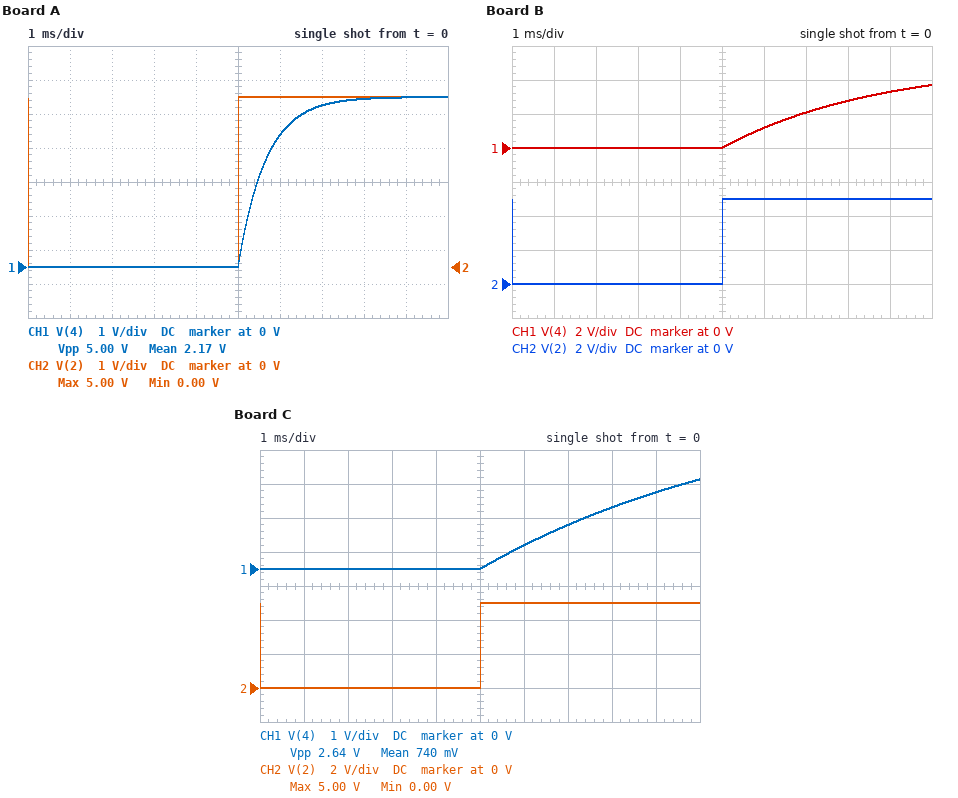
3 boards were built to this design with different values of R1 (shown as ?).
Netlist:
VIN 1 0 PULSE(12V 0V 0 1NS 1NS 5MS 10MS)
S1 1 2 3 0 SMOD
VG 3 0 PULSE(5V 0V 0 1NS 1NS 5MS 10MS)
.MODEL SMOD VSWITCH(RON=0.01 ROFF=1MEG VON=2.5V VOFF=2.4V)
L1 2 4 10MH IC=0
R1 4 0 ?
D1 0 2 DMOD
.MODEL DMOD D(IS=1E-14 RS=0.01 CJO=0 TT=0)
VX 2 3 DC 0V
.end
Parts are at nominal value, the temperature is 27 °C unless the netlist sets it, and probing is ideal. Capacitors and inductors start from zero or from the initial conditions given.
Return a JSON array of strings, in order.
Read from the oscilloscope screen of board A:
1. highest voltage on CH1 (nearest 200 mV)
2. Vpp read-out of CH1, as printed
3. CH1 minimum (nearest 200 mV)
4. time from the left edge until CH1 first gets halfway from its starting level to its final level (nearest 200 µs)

["5.0 V", "5.00 V", "0 V", "5.4 ms"]
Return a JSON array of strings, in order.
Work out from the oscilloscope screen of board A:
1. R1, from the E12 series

["15 Ω"]
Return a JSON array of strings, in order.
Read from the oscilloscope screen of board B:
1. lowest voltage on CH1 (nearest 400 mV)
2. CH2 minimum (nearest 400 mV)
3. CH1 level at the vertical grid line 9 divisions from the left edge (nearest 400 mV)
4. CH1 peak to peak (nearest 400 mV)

["0 V", "0 V", "3.2 V", "3.6 V"]
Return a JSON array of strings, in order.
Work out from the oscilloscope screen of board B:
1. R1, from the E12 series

["2.7 Ω"]
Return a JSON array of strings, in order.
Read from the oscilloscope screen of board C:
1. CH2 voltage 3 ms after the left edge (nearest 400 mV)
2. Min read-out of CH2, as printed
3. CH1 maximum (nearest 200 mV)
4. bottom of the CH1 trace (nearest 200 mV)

["0 V", "0.00 V", "2.6 V", "0 V"]
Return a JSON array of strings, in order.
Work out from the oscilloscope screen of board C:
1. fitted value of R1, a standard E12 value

["1.5 Ω"]
